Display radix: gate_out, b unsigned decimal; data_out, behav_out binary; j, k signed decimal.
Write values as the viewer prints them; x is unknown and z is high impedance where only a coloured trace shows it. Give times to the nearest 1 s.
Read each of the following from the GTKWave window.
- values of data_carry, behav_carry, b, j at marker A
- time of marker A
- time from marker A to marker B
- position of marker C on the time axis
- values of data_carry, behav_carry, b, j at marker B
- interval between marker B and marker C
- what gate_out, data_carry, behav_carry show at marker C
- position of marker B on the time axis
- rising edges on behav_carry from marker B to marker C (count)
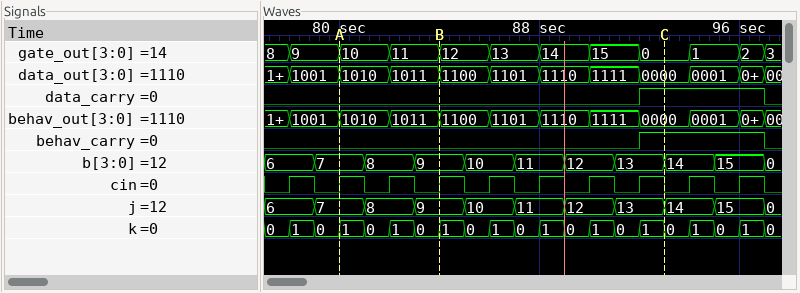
data_carry=0, behav_carry=0, b=7, j=7
80 s
4 s
93 s
data_carry=0, behav_carry=0, b=9, j=9
9 s
gate_out=0, data_carry=1, behav_carry=1
84 s
1
